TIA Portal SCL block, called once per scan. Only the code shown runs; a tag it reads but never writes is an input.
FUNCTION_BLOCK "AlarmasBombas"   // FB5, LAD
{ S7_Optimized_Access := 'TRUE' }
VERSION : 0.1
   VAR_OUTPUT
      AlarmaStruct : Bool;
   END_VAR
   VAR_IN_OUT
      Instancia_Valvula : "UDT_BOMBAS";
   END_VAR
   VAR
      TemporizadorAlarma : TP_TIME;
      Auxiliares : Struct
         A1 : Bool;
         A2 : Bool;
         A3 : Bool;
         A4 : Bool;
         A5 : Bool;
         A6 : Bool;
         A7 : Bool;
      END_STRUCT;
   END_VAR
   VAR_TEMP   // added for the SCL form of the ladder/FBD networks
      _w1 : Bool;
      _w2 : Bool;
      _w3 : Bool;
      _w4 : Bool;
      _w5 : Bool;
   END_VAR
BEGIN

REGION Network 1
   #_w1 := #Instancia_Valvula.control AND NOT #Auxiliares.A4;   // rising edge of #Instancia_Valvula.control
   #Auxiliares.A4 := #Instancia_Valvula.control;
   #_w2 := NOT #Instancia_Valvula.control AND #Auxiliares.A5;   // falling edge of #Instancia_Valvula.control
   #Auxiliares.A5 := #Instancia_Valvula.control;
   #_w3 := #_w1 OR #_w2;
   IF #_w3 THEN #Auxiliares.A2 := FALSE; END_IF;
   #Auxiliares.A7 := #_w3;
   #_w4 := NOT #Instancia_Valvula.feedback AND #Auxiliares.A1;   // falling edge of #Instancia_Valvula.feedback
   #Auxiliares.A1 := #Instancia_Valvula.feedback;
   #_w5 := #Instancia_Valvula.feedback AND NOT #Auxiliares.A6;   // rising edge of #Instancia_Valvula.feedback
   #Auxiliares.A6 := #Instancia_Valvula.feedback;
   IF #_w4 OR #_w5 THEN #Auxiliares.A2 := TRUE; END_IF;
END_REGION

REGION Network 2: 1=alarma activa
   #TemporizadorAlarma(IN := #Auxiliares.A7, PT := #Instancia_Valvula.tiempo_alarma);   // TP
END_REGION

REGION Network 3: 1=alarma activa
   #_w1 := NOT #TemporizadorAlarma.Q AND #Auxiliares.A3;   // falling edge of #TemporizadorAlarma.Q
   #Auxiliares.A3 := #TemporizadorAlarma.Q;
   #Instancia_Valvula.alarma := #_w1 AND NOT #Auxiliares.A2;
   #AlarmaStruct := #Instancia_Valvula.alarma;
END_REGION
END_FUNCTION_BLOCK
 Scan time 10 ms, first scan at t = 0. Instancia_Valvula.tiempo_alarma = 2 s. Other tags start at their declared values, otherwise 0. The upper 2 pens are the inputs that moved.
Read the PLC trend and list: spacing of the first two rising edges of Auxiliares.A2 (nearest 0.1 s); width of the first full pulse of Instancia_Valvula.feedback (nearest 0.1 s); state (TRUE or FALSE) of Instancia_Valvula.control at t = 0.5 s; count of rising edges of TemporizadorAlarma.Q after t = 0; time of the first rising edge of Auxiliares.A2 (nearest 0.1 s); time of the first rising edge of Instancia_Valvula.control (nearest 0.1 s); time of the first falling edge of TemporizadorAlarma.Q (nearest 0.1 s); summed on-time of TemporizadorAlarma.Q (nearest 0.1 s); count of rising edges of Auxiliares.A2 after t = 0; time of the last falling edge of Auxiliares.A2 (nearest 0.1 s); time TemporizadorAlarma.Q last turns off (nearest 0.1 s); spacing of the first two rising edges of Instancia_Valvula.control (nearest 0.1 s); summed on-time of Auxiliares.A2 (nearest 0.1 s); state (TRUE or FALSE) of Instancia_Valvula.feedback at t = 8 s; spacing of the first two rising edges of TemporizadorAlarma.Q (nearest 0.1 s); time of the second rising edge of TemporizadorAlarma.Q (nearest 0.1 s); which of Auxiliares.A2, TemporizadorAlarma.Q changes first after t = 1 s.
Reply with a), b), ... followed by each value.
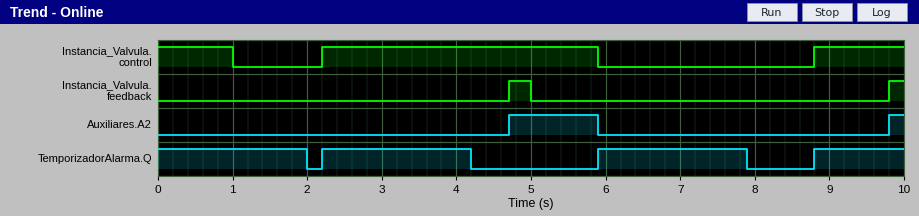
a) 5.1 s
b) 0.3 s
c) TRUE
d) 3
e) 4.7 s
f) 2.2 s
g) 2.0 s
h) 7.2 s
i) 2
j) 5.9 s
k) 7.9 s
l) 6.6 s
m) 1.4 s
n) FALSE
o) 3.7 s
p) 5.9 s
q) TemporizadorAlarma.Q
